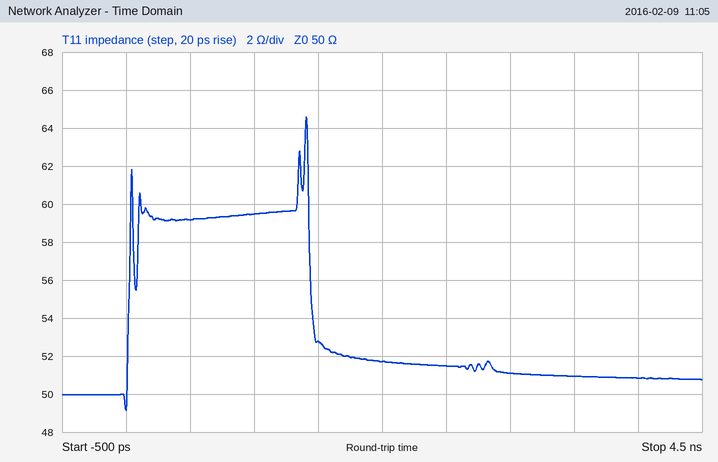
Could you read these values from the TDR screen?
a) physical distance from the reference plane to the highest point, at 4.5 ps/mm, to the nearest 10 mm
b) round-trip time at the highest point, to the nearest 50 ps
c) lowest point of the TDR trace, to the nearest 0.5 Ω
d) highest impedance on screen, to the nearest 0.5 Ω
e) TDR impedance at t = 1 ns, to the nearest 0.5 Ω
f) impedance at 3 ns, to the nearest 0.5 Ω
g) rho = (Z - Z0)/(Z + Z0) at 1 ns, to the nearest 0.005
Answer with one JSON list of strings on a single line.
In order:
["160 mm", "1.40 ns", "49.0 Ω", "64.5 Ω", "59.5 Ω", "51.0 Ω", "+0.085"]
